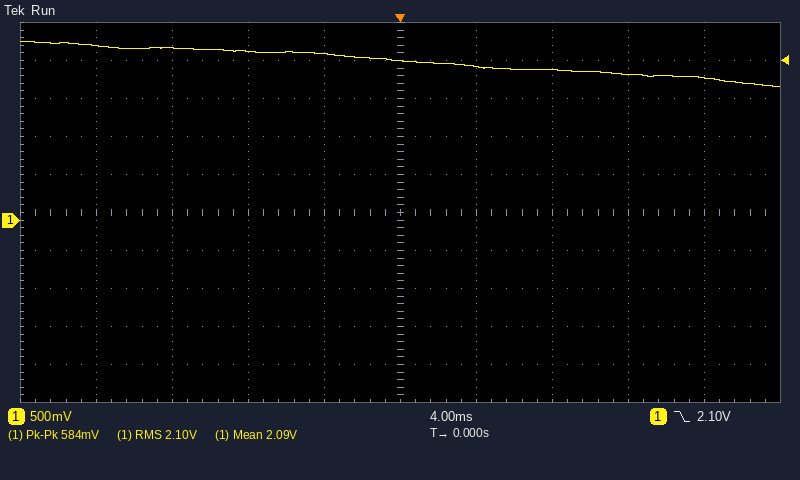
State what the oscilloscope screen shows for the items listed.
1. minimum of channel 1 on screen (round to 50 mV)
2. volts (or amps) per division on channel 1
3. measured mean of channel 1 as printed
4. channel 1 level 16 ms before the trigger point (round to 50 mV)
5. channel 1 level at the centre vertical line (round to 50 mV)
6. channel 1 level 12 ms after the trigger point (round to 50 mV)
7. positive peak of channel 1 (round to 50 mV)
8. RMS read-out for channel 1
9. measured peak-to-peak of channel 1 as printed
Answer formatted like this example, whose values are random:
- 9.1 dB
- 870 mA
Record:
- 1.75 V
- 500 mV
- 2.09 V
- 2.30 V
- 2.10 V
- 1.90 V
- 2.35 V
- 2.10 V
- 584 mV
